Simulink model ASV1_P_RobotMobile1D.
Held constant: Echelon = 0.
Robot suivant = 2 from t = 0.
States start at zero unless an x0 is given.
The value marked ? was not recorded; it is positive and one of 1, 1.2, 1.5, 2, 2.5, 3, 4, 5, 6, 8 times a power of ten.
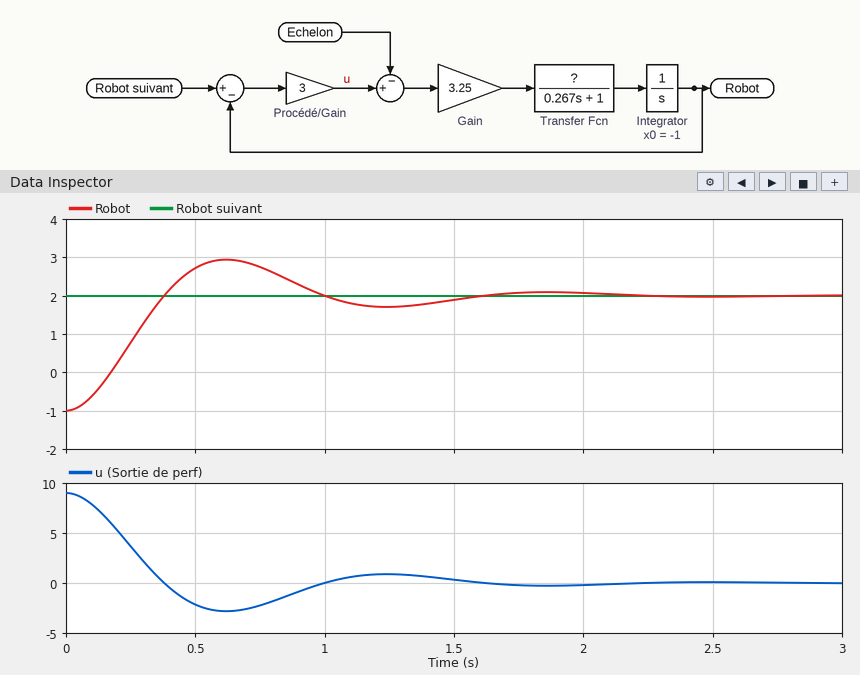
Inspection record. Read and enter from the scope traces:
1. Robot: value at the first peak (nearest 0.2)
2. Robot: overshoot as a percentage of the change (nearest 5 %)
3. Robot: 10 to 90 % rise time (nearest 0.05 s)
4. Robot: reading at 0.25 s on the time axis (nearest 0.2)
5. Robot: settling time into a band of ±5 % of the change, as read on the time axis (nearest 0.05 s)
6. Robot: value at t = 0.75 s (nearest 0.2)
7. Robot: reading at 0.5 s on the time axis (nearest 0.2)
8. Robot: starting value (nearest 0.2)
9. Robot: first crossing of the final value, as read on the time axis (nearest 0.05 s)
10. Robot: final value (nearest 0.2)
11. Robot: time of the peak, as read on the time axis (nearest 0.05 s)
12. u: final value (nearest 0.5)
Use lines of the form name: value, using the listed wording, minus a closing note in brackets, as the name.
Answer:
Robot: value at the first peak: 3.0
Robot: overshoot as a percentage of the change: 30 %
Robot: 10 to 90 % rise time: 0.25 s
Robot: reading at 0.25 s on the time axis: 0.8
Robot: settling time into a band of ±5 % of the change, as read on the time axis: 1.45 s
Robot: value at t = 0.75 s: 2.8
Robot: reading at 0.5 s on the time axis: 2.8
Robot: starting value: -1.0
Robot: first crossing of the final value, as read on the time axis: 0.40 s
Robot: final value: 2.0
Robot: time of the peak, as read on the time axis: 0.60 s
u: final value: 0.0
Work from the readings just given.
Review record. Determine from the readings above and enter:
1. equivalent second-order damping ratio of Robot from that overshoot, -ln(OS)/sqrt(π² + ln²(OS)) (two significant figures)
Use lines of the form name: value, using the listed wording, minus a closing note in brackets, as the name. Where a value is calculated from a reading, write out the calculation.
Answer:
equivalent second-order damping ratio of Robot from that overshoot, -ln(OS)/sqrt(π² + ln²(OS)): ln(0.3) = -1.204; 1.204 / sqrt(9.870 + 1.450) = 0.36
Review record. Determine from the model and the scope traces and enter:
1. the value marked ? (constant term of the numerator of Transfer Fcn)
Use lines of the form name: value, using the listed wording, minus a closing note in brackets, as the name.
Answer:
the value marked ?: 0.8
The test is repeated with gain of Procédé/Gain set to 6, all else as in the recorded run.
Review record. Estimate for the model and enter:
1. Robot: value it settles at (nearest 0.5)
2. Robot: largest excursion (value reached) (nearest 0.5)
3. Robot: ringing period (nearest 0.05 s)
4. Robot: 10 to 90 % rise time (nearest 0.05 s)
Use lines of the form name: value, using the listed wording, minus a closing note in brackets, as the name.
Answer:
Robot: value it settles at: 2.0
Robot: largest excursion (value reached): 3.5
Robot: ringing period: 0.85 s
Robot: 10 to 90 % rise time: 0.15 s
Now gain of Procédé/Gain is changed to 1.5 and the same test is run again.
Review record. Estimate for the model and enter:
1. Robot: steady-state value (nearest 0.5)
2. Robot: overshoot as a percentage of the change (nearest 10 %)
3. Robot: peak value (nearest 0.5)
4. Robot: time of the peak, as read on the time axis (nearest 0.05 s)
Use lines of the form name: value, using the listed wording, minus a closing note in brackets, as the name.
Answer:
Robot: steady-state value: 2.0
Robot: overshoot as a percentage of the change: 20 %
Robot: peak value: 2.5
Robot: time of the peak, as read on the time axis: 0.95 s
